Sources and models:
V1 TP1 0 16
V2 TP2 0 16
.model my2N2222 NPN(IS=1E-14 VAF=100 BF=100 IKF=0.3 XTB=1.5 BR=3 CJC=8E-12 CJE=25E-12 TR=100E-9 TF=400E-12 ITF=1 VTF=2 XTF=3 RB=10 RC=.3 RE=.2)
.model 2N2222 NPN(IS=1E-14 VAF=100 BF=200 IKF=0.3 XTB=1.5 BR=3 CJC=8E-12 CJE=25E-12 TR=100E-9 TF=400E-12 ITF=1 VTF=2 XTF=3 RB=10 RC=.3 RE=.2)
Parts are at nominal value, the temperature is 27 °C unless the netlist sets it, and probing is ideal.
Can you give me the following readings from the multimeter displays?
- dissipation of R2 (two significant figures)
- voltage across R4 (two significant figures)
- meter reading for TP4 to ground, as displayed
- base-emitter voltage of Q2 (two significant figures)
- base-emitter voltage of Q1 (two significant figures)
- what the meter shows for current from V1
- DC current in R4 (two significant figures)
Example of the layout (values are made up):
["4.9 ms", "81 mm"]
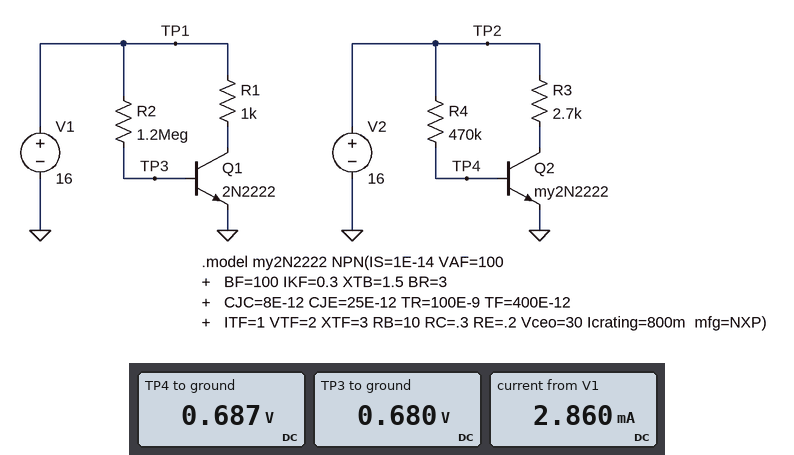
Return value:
["200 µW", "15 V", "0.687 V", "690 mV", "680 mV", "2.860 mA", "33 µA"]
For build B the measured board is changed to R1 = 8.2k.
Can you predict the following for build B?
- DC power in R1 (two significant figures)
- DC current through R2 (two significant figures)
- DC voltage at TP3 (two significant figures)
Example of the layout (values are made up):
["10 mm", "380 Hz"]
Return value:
["31 mW", "13 µA", "670 mV"]
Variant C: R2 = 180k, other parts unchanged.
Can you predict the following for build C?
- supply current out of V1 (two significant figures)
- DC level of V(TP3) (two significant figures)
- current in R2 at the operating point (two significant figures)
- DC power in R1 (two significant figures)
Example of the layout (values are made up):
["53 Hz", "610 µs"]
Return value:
["16 mA", "730 mV", "85 µA", "250 mW"]
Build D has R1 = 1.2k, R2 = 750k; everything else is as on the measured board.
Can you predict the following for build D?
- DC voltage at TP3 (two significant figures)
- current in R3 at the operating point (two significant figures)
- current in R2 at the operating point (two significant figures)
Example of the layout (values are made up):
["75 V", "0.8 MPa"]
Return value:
["690 mV", "3.4 mA", "20 µA"]
